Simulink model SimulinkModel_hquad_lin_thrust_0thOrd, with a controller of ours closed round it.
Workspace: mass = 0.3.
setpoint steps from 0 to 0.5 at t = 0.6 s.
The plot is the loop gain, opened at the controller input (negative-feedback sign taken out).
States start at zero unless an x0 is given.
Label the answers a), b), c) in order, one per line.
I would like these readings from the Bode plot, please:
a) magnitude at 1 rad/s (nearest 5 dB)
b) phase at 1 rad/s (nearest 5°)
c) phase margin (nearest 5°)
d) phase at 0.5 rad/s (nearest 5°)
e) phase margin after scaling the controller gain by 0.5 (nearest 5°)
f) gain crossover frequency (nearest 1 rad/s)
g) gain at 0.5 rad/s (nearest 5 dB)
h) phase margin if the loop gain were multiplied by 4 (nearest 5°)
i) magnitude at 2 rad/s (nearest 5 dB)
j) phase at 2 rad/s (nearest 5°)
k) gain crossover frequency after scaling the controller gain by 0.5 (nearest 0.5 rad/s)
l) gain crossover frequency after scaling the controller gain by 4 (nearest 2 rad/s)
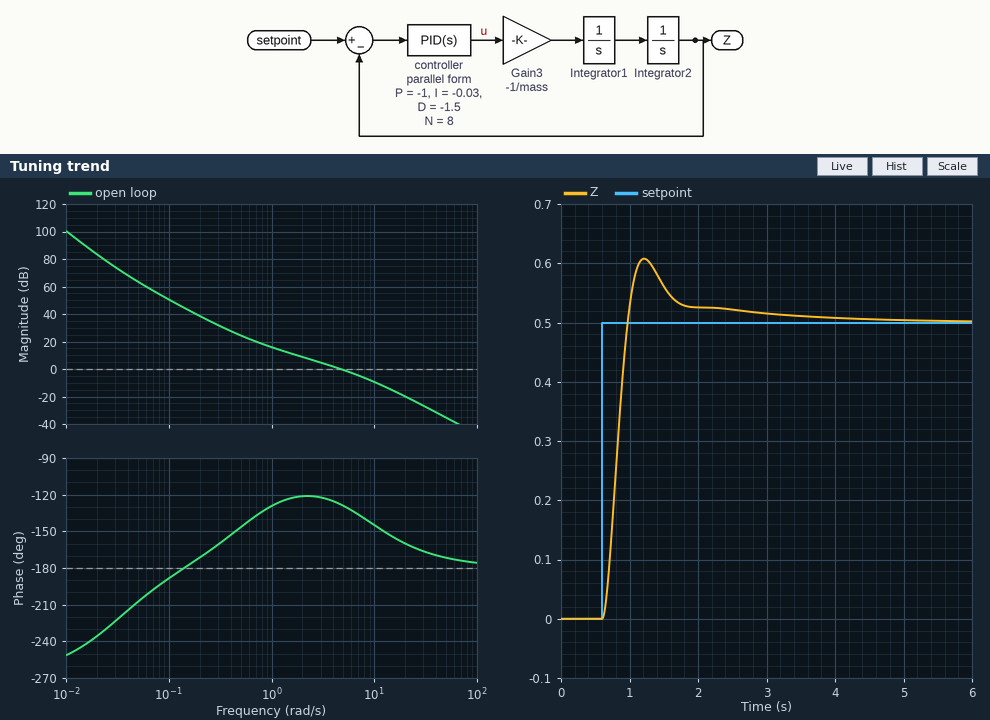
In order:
a) 15 dB
b) -130°
c) 50°
d) -145°
e) 60°
f) 5 rad/s
g) 25 dB
h) 30°
i) 10 dB
j) -120°
k) 2.5 rad/s
l) 12 rad/s
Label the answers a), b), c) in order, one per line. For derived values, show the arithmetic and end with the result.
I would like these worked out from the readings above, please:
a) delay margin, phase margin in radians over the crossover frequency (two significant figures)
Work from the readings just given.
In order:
a) 50 × π / 180 / 5 = 0.17 s
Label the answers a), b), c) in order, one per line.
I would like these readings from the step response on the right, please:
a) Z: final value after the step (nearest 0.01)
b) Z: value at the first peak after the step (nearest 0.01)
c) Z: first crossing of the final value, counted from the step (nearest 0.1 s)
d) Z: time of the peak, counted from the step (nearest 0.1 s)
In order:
a) 0.50
b) 0.61
c) 0.4 s
d) 0.6 s
